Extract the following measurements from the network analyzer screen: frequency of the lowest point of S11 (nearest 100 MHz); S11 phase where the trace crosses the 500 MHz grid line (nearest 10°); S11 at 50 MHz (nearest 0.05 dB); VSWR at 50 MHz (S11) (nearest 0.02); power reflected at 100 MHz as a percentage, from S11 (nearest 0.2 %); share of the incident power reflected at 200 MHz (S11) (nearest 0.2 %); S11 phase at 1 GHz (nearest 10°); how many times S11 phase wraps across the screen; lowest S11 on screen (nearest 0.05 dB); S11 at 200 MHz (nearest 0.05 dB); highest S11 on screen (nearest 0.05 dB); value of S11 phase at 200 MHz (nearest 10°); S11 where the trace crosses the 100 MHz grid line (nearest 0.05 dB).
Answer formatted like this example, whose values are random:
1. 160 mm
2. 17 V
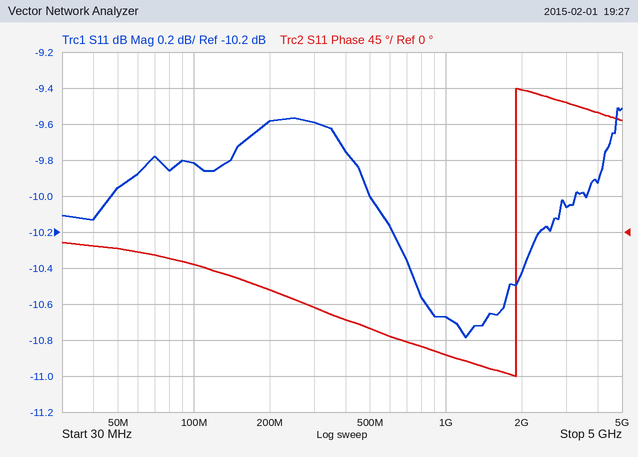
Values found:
1. 1.2 GHz
2. -120°
3. -9.95 dB
4. 1.94
5. 10.4 %
6. 11.0 %
7. -150°
8. 1
9. -10.80 dB
10. -9.60 dB
11. -9.50 dB
12. -70°
13. -9.80 dB
